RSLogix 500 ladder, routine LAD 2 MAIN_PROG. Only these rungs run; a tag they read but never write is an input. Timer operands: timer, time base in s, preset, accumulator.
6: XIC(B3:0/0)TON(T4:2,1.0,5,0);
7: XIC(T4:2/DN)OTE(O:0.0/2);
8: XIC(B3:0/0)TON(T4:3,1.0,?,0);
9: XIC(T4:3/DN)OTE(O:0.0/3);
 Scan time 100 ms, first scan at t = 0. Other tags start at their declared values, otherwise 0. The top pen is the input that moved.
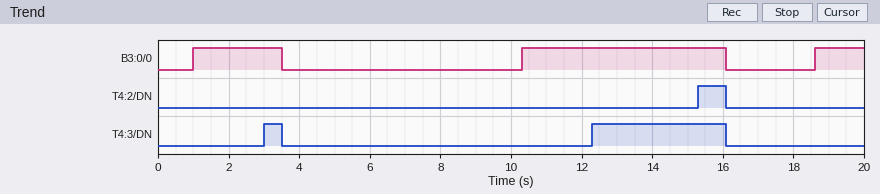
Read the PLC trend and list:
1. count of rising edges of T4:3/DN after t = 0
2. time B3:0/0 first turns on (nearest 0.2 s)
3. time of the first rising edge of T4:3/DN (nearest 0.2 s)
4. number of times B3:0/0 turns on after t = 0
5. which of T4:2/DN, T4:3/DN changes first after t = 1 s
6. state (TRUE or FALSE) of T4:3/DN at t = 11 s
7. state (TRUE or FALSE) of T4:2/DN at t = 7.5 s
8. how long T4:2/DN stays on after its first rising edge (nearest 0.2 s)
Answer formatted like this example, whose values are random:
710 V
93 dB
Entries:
2
1.0 s
3.0 s
3
T4:3/DN
FALSE
FALSE
0.8 s
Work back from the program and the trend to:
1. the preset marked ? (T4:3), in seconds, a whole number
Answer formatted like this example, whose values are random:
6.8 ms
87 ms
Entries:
2 s
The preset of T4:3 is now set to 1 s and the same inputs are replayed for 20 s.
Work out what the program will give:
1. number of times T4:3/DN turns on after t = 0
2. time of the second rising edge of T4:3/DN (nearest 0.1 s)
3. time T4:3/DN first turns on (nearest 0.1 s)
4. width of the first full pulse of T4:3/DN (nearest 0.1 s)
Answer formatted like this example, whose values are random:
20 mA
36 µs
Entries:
3
11.3 s
2.0 s
1.5 s
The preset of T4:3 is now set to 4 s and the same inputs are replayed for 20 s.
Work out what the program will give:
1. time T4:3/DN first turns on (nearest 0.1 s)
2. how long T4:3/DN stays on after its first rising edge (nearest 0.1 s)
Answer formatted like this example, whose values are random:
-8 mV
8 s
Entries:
14.3 s
1.8 s
